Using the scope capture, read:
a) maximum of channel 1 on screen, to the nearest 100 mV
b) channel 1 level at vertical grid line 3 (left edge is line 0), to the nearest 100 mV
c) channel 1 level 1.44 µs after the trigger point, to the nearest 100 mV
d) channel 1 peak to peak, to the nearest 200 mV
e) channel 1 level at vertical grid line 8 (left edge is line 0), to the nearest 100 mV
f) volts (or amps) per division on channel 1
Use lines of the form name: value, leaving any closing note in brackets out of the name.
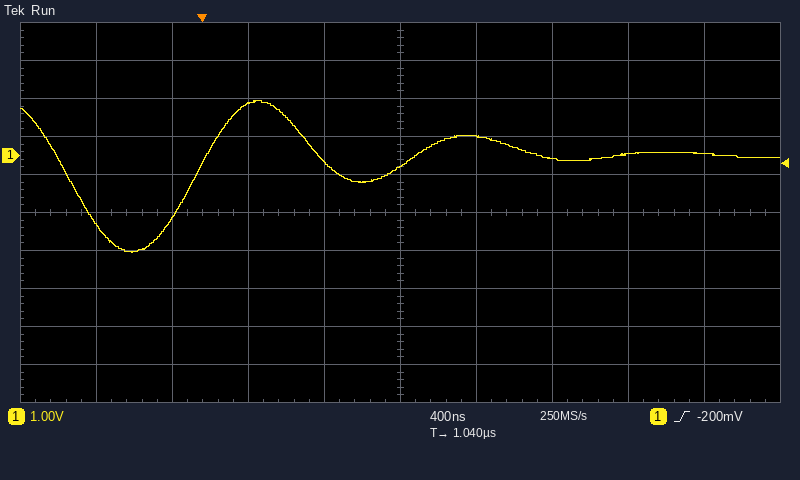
maximum of channel 1 on screen, to the nearest 100 mV: 1.4 V
channel 1 level at vertical grid line 3 (left edge is line 0), to the nearest 100 mV: 1.4 V
channel 1 level 1.44 µs after the trigger point, to the nearest 100 mV: 500 mV
channel 1 peak to peak, to the nearest 200 mV: 4.0 V
channel 1 level at vertical grid line 8 (left edge is line 0), to the nearest 100 mV: 0.0 V
volts (or amps) per division on channel 1: 1 V
